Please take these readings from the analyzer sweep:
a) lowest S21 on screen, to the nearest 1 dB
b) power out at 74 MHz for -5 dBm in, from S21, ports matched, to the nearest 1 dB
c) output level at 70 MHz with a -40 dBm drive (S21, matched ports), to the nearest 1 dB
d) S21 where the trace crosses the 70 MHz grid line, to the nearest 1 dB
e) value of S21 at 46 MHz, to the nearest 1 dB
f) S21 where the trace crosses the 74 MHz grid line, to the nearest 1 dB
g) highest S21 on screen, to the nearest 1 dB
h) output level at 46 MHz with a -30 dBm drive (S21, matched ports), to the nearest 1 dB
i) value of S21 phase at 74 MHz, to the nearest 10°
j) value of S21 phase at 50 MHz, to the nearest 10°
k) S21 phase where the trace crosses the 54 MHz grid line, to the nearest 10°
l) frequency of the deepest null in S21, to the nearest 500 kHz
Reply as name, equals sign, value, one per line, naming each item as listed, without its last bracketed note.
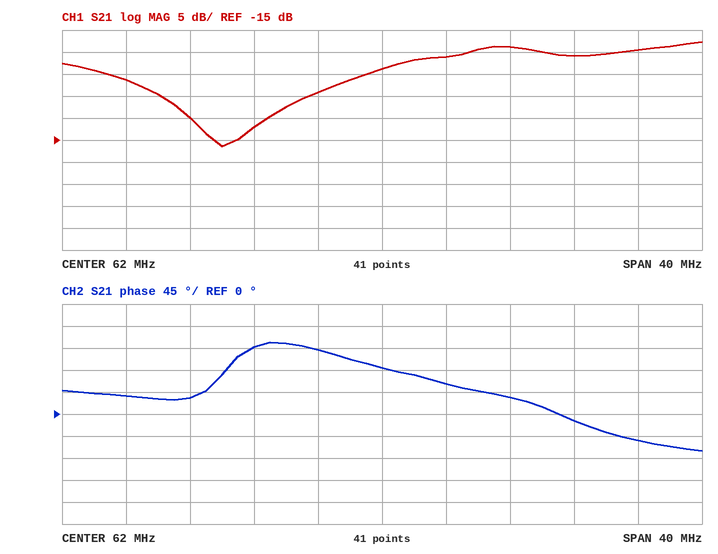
lowest S21 on screen, to the nearest 1 dB = -16 dB
power out at 74 MHz for -5 dBm in, from S21, ports matched, to the nearest 1 dB = -1 dBm
output level at 70 MHz with a -40 dBm drive (S21, matched ports), to the nearest 1 dB = -34 dBm
S21 where the trace crosses the 70 MHz grid line, to the nearest 1 dB = 6 dB
value of S21 at 46 MHz, to the nearest 1 dB = -1 dB
S21 where the trace crosses the 74 MHz grid line, to the nearest 1 dB = 4 dB
highest S21 on screen, to the nearest 1 dB = 7 dB
output level at 46 MHz with a -30 dBm drive (S21, matched ports), to the nearest 1 dB = -31 dBm
value of S21 phase at 74 MHz, to the nearest 10° = -10°
value of S21 phase at 50 MHz, to the nearest 10° = 30°
S21 phase where the trace crosses the 54 MHz grid line, to the nearest 10° = 140°
frequency of the deepest null in S21, to the nearest 500 kHz = 52.0 MHz
